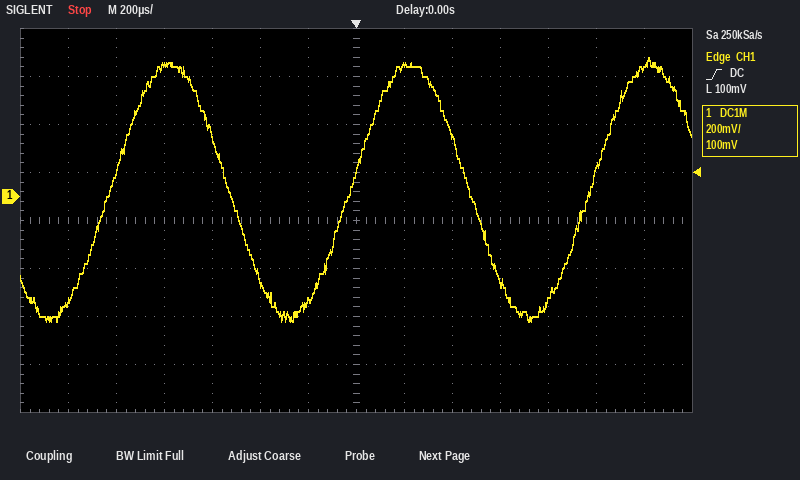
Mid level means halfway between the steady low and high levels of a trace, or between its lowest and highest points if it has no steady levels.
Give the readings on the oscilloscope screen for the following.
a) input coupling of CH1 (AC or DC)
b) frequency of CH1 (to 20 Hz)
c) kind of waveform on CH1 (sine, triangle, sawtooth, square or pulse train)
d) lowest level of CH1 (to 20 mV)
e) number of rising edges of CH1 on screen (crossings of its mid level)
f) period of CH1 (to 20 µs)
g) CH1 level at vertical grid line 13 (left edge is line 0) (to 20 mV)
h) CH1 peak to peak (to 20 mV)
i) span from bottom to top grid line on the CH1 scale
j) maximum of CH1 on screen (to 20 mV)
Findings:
DC
1.00 kHz
sine
-520 mV
3
1.00 ms
540 mV
1.10 V
1.6 V
580 mV
